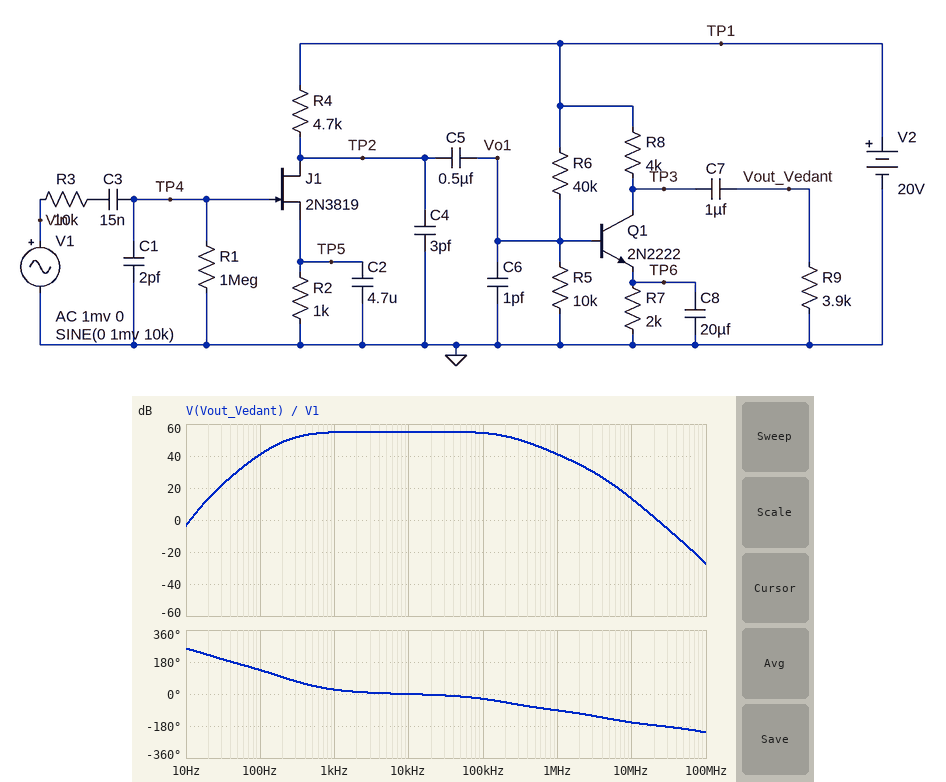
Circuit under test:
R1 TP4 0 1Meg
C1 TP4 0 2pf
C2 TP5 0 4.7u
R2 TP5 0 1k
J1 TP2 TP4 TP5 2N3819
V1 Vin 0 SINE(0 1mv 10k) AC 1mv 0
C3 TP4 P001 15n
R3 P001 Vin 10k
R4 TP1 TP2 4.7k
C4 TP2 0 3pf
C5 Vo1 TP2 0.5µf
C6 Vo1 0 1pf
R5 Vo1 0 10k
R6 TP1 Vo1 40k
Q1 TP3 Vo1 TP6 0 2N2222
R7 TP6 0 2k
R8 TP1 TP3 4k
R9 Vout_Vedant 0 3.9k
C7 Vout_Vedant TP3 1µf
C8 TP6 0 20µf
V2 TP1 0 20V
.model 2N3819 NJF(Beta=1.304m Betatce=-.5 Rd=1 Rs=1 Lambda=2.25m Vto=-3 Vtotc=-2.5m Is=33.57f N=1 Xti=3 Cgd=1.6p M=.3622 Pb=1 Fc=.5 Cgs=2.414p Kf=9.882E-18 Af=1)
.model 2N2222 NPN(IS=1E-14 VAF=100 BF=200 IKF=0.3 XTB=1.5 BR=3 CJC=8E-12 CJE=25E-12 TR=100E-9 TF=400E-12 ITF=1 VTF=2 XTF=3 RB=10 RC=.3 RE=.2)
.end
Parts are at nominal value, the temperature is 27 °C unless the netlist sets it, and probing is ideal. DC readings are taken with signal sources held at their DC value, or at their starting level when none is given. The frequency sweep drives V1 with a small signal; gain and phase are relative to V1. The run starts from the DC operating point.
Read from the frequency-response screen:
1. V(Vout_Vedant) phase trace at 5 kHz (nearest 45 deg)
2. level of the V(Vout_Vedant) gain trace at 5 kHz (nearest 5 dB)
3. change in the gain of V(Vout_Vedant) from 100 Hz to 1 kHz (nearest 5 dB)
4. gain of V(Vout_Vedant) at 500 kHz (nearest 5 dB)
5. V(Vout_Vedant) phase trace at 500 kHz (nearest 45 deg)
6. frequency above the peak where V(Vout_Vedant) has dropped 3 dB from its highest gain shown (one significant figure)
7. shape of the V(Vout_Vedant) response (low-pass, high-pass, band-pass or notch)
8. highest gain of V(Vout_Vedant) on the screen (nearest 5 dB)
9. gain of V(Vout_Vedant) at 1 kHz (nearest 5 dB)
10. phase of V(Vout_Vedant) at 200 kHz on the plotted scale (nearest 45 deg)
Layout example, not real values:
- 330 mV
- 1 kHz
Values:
- 0 deg
- 55 dB
- 15 dB
- 45 dB
- -90 deg
- 200 kHz
- band-pass
- 55 dB
- 55 dB
- -45 deg
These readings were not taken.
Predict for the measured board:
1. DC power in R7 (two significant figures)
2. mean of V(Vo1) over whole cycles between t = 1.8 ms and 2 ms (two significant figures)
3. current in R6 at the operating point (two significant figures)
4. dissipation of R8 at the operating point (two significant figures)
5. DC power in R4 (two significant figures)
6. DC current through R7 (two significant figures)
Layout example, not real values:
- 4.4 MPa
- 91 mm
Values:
- 5.4 mW
- 3.9 V
- 400 µA
- 11 mW
- 16 mW
- 1.6 mA
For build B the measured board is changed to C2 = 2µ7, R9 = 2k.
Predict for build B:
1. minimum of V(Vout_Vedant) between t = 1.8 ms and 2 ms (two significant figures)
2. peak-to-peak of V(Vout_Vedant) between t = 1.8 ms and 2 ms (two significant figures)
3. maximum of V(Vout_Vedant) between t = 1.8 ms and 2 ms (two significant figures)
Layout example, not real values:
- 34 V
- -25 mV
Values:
- -400 mV
- 790 mV
- 390 mV
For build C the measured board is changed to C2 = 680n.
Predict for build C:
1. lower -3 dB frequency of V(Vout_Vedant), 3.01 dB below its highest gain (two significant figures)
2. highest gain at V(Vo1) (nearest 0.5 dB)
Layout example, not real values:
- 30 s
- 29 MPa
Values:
- 980 Hz
- 14.0 dB
